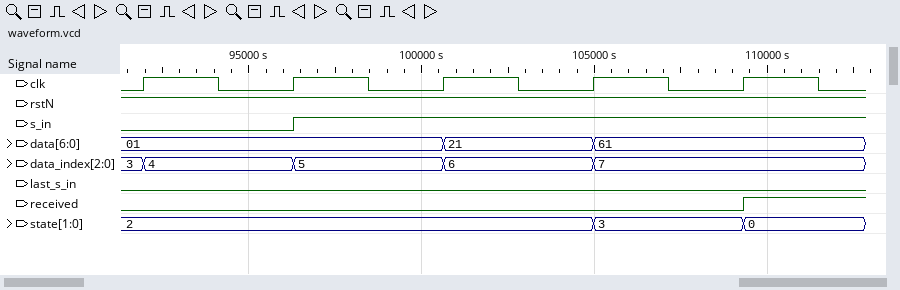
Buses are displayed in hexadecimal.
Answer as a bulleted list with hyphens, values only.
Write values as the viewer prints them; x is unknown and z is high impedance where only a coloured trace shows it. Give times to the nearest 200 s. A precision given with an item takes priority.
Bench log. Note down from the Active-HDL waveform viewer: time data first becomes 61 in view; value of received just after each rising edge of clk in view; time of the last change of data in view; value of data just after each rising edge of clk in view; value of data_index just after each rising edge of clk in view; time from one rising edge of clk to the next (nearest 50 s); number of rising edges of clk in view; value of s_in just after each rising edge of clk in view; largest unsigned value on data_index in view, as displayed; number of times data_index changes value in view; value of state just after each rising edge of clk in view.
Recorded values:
- 105000 s
- 0 0 0 0 1
- 105000 s
- 01, 01, 21, 61, 61
- 4, 5, 6, 7, 7
- 4350 s
- 5
- 0 1 1 1 1
- 7
- 4
- 2, 2, 2, 3, 0
